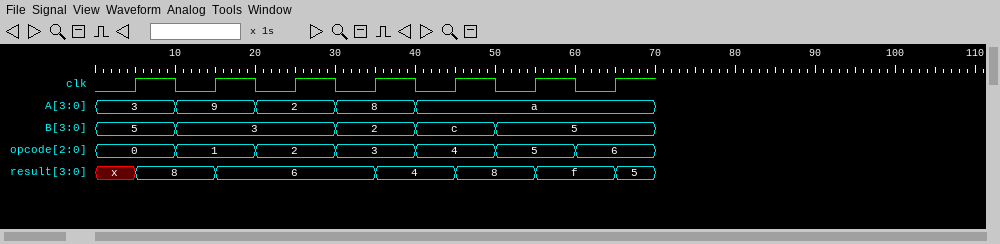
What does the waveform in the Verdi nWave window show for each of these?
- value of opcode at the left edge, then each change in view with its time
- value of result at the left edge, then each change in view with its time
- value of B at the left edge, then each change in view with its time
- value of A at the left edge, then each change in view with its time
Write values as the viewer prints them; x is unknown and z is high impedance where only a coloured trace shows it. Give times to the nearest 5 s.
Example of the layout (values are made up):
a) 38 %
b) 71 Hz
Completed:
a) 0, 1 at 10 s, 2 at 20 s, 3 at 30 s, 4 at 40 s, 5 at 50 s, 6 at 60 s
b) x, 8 at 5 s, 6 at 15 s, 4 at 35 s, 8 at 45 s, f at 55 s, 5 at 65 s
c) 5, 3 at 10 s, 2 at 30 s, c at 40 s, 5 at 50 s
d) 3, 9 at 10 s, 2 at 20 s, 8 at 30 s, a at 40 s
